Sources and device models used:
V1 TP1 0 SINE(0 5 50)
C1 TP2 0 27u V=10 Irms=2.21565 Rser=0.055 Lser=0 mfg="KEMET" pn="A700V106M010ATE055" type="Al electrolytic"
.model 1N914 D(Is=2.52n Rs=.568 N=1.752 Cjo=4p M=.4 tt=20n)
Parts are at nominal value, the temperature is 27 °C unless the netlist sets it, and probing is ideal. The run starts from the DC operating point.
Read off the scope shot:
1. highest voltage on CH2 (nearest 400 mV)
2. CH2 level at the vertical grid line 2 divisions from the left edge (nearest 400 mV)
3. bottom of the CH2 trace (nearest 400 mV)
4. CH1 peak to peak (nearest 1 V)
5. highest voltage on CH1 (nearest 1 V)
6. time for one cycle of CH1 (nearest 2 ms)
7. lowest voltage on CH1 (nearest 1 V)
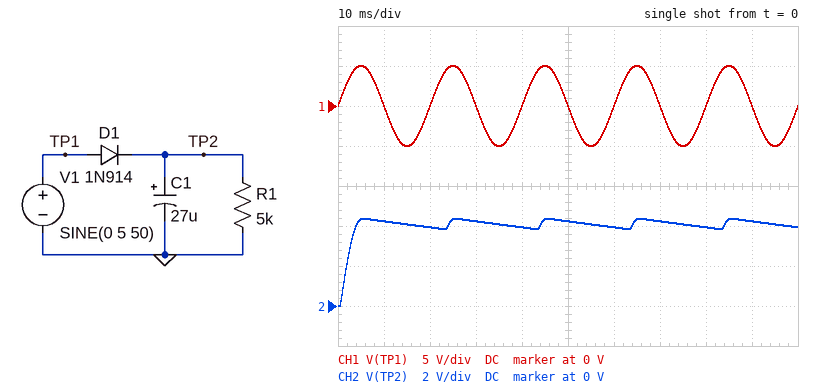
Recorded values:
4.4 V
4.0 V
0 V
10 V
5 V
20 ms
-5 V
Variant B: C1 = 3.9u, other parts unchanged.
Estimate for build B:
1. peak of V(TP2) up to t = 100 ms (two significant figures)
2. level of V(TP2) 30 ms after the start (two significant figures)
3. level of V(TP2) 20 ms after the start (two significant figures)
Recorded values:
4.4 V
3.5 V
2.1 V
